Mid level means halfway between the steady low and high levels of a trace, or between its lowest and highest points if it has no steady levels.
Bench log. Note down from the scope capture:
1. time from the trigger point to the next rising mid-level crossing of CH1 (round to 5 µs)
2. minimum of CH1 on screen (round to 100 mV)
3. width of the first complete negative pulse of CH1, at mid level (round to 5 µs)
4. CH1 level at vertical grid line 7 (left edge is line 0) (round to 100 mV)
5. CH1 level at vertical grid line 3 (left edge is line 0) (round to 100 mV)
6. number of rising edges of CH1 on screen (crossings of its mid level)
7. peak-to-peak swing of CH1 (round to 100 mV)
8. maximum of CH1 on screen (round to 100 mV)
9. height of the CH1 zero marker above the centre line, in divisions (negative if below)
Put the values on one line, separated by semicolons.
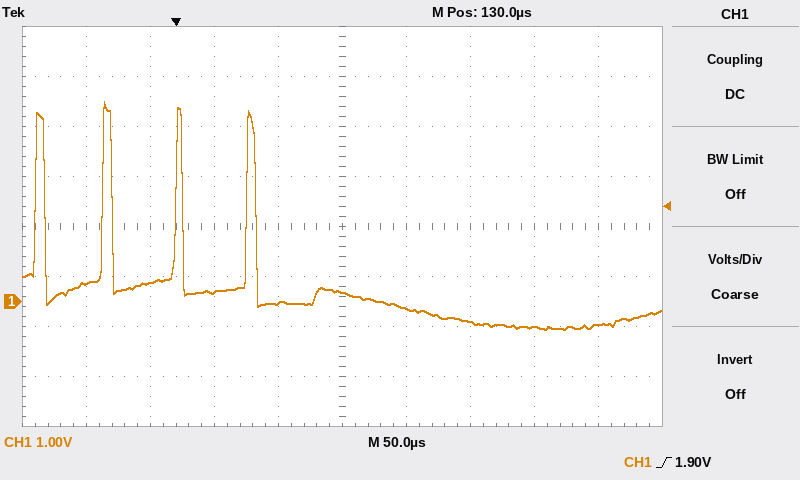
55 µs; -600 mV; 45 µs; -400 mV; 200 mV; 4; 4.6 V; 4.0 V; -1.5 div
